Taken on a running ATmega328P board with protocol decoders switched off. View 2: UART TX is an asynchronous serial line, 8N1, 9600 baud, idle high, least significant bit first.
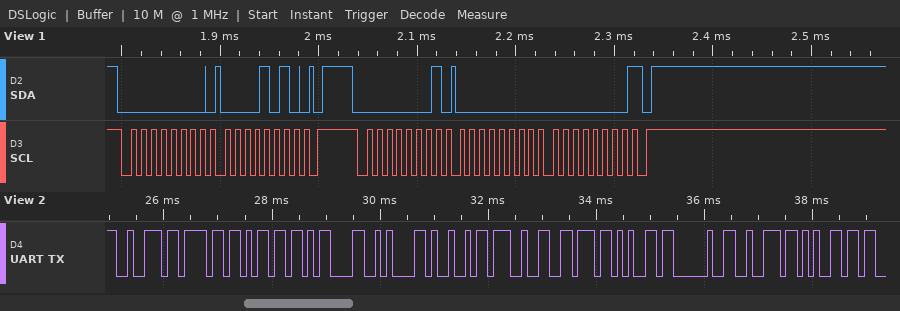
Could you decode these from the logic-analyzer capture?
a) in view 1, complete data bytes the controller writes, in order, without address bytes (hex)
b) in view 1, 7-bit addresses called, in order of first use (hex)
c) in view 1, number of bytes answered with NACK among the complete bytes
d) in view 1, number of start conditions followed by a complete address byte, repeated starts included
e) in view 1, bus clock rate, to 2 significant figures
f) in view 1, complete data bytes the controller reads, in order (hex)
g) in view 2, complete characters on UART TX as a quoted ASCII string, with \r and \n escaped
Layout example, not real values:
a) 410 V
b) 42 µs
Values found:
a) 0A
b) 0x00
c) 1
d) 2
e) 100 kHz
f) 00 00
g) "rom\r\nI've re"
